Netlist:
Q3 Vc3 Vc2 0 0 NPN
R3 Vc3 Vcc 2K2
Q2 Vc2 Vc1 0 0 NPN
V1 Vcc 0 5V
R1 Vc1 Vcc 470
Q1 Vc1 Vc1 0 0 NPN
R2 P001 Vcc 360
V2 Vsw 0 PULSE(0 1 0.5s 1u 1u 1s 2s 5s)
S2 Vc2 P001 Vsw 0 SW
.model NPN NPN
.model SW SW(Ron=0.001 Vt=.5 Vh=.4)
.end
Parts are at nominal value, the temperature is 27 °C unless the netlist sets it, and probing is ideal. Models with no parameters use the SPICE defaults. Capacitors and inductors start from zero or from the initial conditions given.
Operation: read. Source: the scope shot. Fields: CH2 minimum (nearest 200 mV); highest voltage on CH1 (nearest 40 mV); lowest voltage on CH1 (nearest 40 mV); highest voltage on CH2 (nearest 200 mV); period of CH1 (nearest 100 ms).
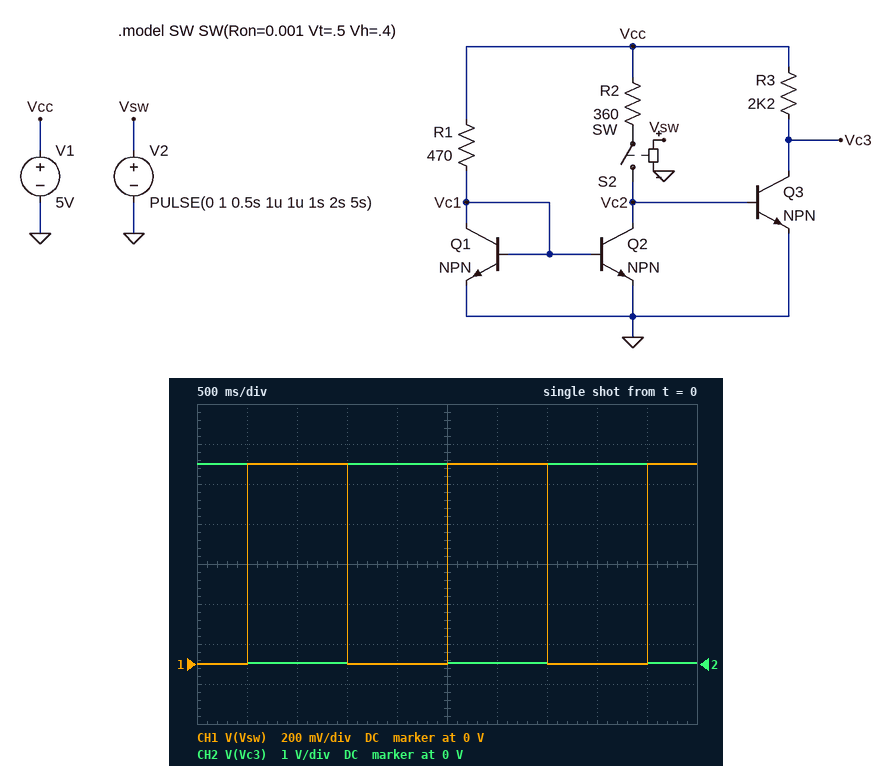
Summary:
0 V
1.00 V
0 V
5.0 V
2.0 s
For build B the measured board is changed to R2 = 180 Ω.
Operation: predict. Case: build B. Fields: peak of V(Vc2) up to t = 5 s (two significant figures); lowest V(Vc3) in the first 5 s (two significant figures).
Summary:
860 mV
20 mV
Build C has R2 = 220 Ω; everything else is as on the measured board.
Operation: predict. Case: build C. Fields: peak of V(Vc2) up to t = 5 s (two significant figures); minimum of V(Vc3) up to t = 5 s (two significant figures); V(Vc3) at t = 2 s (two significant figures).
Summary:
850 mV
21 mV
5.0 V
